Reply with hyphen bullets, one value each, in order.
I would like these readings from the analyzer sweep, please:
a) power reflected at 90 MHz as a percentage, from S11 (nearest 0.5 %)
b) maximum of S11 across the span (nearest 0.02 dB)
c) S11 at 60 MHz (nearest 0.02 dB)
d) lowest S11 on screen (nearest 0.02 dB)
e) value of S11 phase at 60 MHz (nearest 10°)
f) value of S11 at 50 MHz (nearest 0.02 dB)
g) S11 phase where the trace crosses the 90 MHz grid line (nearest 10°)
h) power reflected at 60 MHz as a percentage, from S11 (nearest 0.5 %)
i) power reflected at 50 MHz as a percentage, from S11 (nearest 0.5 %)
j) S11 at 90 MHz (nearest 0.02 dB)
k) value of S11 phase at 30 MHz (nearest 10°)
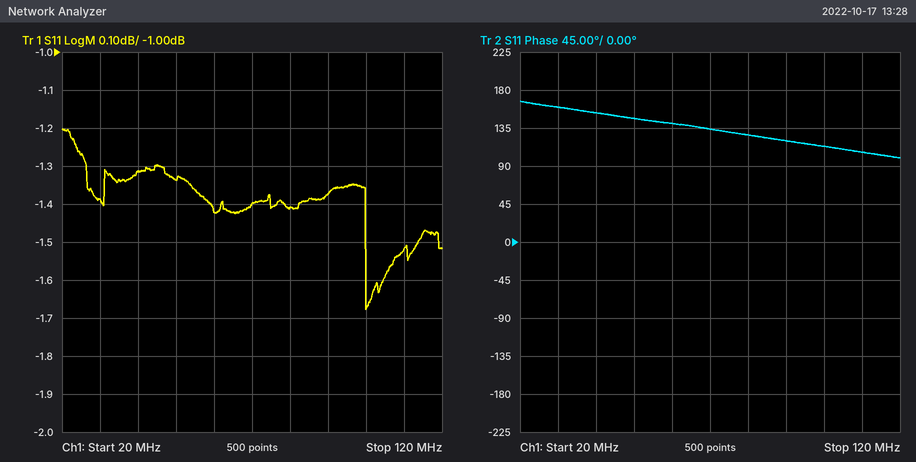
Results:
- 73.0 %
- -1.20 dB
- -1.42 dB
- -1.68 dB
- 140°
- -1.34 dB
- 120°
- 72.0 %
- 73.5 %
- -1.38 dB
- 160°
